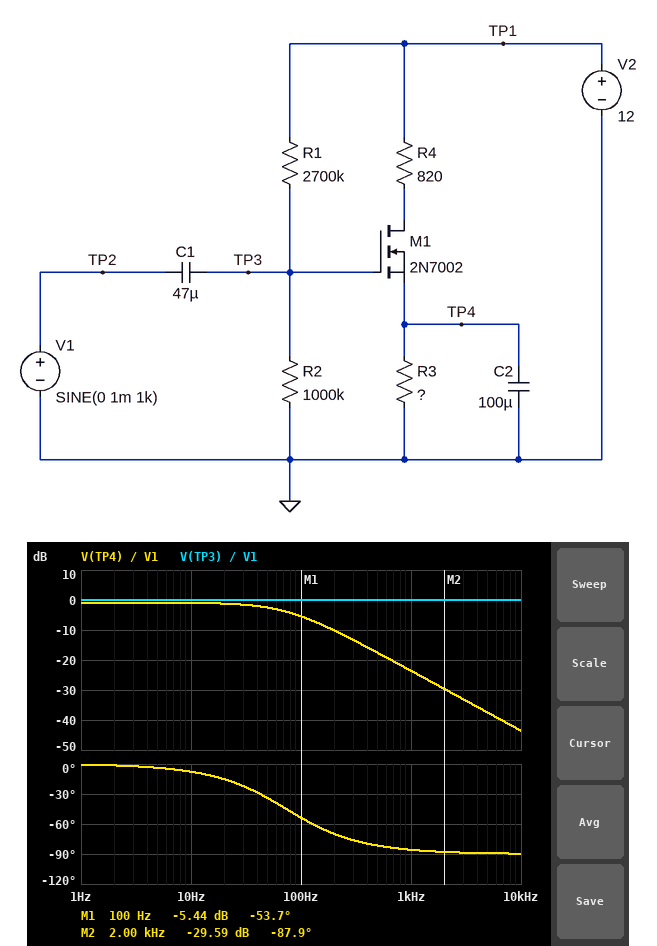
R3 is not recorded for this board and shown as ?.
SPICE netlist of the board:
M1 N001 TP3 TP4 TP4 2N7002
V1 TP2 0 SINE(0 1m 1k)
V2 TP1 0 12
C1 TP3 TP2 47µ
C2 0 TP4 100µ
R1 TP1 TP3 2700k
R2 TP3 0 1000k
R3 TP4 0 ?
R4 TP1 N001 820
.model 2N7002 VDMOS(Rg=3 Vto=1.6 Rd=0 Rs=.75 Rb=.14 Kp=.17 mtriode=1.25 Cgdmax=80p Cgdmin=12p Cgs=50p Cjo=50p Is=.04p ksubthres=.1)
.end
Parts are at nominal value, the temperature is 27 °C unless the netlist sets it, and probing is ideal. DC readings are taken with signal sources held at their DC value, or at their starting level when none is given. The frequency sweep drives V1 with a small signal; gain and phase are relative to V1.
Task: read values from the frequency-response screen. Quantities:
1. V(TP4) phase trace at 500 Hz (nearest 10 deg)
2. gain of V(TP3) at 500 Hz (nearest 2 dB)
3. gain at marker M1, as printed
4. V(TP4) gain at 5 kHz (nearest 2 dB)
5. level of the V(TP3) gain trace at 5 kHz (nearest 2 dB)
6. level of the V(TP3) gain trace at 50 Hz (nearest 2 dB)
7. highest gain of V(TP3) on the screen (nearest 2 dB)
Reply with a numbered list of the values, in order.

1. -80 deg
2. 0 dB
3. -5.44 dB
4. -38 dB
5. 0 dB
6. 0 dB
7. 0 dB
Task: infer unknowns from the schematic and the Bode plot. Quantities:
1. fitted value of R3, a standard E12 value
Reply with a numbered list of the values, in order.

1. 220 Ω
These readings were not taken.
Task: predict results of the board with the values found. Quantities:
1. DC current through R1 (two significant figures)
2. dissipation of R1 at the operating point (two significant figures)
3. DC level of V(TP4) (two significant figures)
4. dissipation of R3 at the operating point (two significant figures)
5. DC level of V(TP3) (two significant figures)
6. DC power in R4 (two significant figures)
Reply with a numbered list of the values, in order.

1. 3.2 µA
2. 28 µW
3. 1.4 V
4. 8.6 mW
5. 3.2 V
6. 32 mW
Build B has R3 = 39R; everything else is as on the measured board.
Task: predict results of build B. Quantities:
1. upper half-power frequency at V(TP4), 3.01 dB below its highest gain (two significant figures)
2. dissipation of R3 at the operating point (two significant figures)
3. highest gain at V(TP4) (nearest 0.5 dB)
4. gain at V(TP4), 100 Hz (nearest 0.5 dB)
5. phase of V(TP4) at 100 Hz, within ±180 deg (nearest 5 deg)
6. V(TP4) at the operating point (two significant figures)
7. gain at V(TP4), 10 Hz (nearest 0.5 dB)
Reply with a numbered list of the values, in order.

1. 43 Hz
2. 7.5 mW
3. -51.0 dB
4. -59.5 dB
5. -65 deg
6. 540 mV
7. -51.5 dB
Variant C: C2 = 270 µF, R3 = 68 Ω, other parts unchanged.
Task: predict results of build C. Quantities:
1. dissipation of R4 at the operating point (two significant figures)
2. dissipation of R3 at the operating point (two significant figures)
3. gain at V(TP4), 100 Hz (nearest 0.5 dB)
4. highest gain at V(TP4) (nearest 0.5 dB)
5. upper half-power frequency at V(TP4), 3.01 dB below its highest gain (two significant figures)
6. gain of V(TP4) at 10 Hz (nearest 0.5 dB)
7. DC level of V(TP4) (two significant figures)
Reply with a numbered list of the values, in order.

1. 150 mW
2. 12 mW
3. -59.0 dB
4. -38.5 dB
5. 9.5 Hz
6. -42.0 dB
7. 910 mV
